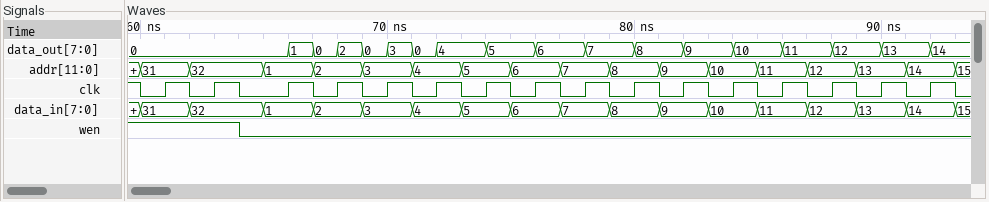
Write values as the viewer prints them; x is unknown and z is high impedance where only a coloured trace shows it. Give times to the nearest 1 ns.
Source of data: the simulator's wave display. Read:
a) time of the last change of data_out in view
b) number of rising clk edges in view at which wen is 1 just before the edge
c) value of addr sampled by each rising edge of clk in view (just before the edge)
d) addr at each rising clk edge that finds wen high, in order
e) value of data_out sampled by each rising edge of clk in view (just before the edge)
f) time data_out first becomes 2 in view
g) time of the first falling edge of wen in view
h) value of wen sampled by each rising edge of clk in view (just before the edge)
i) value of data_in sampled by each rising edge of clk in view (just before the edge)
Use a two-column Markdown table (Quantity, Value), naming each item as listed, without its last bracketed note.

| Quantity | Value |
|---|---|
| time of the last change of data_out in view | 92 ns |
| number of rising clk edges in view at which wen is 1 just before the edge | 2 |
| value of addr sampled by each rising edge of clk in view | 31, 32, 1, 2, 3, 4, 5, 6, 7, 8, 9, 10, 11, 12, 13, 14 |
| addr at each rising clk edge that finds wen high, in order | 31, 32 |
| value of data_out sampled by each rising edge of clk in view | 0, 0, 0, 0, 0, 0, 4, 5, 6, 7, 8, 9, 10, 11, 12, 13 |
| time data_out first becomes 2 in view | 68 ns |
| time of the first falling edge of wen in view | 64 ns |
| value of wen sampled by each rising edge of clk in view | 1 1 0 0 0 0 0 0 0 0 0 0 0 0 0 0 |
| value of data_in sampled by each rising edge of clk in view | 31, 32, 1, 2, 3, 4, 5, 6, 7, 8, 9, 10, 11, 12, 13, 14 |
